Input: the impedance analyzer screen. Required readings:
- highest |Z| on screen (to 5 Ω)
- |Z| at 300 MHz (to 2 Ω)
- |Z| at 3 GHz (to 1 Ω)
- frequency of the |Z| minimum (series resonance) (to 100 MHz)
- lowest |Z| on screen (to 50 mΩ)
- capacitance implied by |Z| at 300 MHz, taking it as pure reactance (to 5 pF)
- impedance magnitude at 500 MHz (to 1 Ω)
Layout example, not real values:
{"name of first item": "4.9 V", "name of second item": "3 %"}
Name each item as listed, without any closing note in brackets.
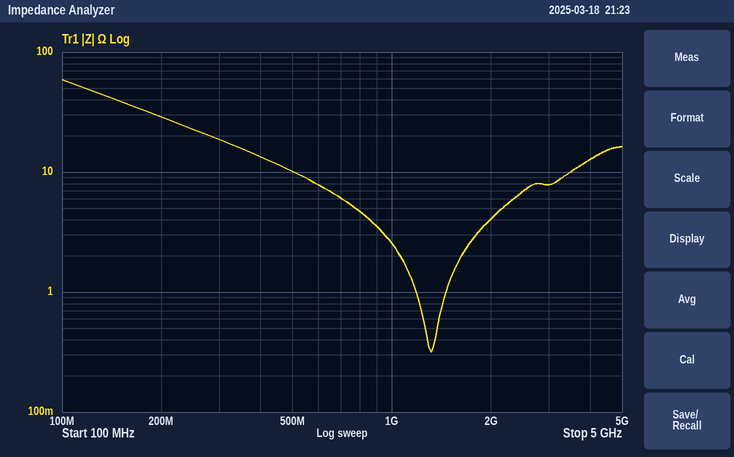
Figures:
{"highest |Z| on screen": "60 Ω", "|Z| at 300 MHz": "18 Ω", "|Z| at 3 GHz": "8 Ω", "frequency of the |Z| minimum (series resonance)": "1.3 GHz", "lowest |Z| on screen": "300 mΩ", "capacitance implied by |Z| at 300 MHz, taking it as pure reactance": "30 pF", "impedance magnitude at 500 MHz": "10 Ω"}
